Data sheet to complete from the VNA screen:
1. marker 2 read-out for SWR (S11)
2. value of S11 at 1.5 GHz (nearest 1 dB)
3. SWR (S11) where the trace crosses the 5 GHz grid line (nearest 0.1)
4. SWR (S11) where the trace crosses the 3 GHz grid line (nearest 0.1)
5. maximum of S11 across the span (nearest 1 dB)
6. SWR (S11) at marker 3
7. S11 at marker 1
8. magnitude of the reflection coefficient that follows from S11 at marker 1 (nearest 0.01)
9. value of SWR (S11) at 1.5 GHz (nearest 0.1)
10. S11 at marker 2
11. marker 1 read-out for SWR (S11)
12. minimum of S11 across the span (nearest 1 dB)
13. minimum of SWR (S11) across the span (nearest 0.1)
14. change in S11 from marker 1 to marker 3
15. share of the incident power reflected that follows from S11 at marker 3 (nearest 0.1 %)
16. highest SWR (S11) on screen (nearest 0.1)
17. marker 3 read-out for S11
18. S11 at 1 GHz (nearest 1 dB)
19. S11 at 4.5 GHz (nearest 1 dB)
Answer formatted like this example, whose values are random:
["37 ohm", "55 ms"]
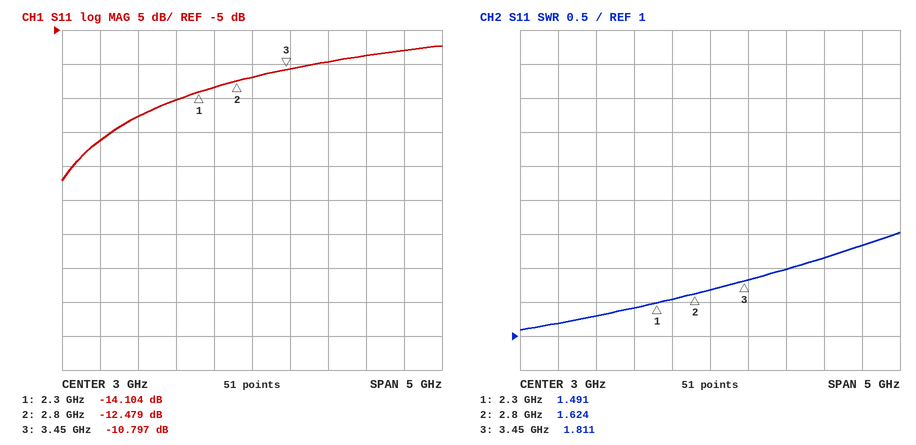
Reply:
["1.624", "-18 dB", "2.3", "1.7", "-7 dB", "1.811", "-14.104 dB", "0.20", "1.3", "-12.479 dB", "1.491", "-27 dB", "1.1", "3.307 dB", "8.3 %", "2.5", "-10.797 dB", "-21 dB", "-9 dB"]
